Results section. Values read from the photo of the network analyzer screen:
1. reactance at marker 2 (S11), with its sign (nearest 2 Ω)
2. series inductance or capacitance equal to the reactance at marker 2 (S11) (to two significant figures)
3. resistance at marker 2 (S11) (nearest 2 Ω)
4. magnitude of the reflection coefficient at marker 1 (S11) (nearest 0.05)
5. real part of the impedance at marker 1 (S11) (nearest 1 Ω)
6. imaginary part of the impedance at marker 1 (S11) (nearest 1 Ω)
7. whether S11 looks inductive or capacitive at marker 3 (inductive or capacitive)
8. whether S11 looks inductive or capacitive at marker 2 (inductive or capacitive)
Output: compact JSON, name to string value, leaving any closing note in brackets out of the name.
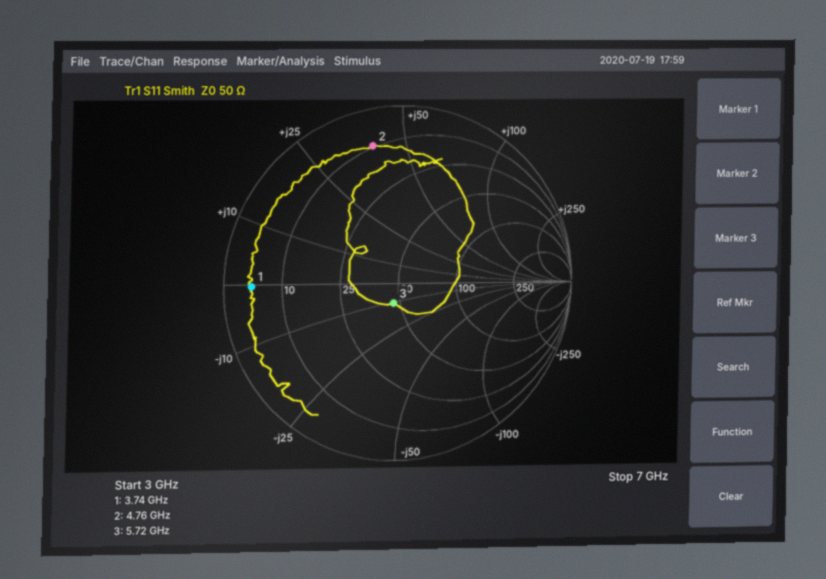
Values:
{"reactance at marker 2 (S11), with its sign": "+40 Ω", "series inductance or capacitance equal to the reactance at marker 2 (S11)": "1.3 nH", "resistance at marker 2 (S11)": "10 Ω", "magnitude of the reflection coefficient at marker 1 (S11)": "0.85", "real part of the impedance at marker 1 (S11)": "4 Ω", "imaginary part of the impedance at marker 1 (S11)": "0 Ω", "whether S11 looks inductive or capacitive at marker 3": "capacitive", "whether S11 looks inductive or capacitive at marker 2": "inductive"}
